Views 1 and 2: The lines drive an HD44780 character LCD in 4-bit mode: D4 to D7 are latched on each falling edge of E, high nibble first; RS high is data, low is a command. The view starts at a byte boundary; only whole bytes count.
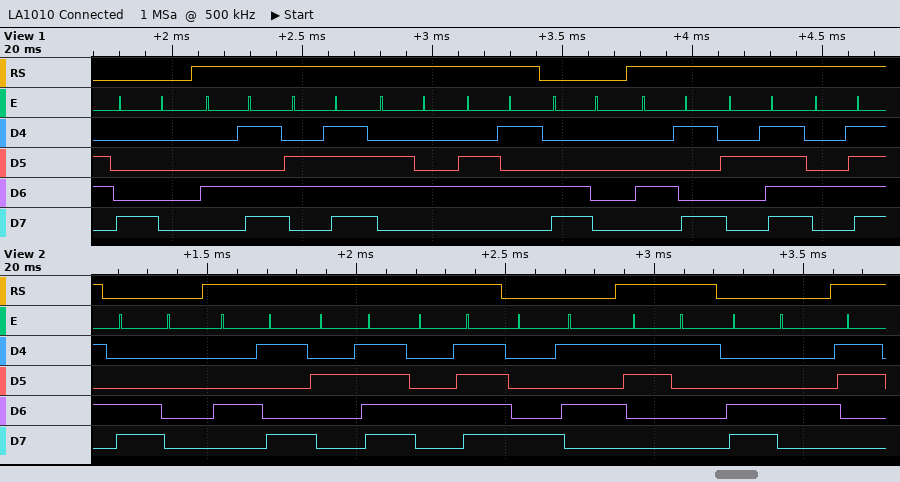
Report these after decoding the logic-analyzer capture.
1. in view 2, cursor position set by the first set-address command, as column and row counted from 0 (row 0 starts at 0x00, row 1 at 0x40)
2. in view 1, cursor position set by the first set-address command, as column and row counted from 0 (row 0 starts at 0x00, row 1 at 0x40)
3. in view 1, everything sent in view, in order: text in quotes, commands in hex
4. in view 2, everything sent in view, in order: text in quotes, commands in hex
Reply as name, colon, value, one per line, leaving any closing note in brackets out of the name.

in view 2, cursor position set by the first set-address command, as column and row counted from 0: column 0, row 1
in view 1, cursor position set by the first set-address command, as column and row counted from 0: column 0, row 0
in view 1, everything sent in view, in order: text in quotes, commands in hex: 0x80 "Mode" 0xC0 "I/O"
in view 2, everything sent in view, in order: text in quotes, commands in hex: 0xC0 "I/O" 0x85 "1" 0xC4
